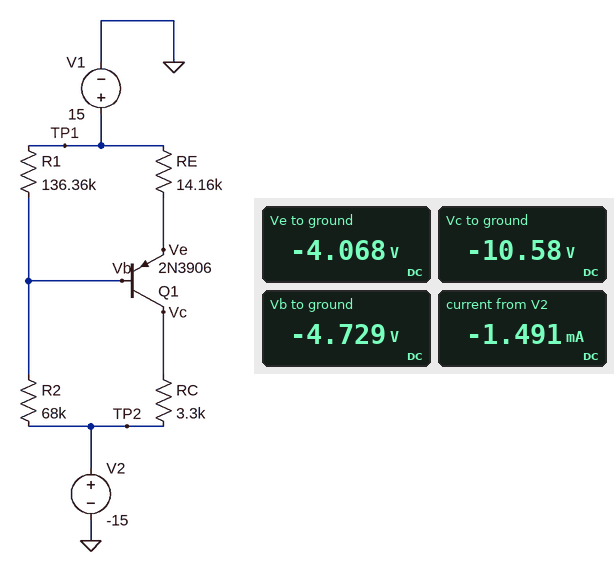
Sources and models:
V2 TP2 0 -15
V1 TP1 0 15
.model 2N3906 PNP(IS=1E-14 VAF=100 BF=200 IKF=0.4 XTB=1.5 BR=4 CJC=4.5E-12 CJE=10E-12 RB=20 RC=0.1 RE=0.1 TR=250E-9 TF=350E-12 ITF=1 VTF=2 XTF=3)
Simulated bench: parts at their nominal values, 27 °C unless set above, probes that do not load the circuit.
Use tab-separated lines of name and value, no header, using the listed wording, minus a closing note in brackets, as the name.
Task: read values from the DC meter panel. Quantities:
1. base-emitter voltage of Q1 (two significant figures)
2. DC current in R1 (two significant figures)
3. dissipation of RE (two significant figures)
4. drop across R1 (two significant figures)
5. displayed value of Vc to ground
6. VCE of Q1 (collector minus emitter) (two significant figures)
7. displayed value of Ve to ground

base-emitter voltage of Q1	-660 mV
DC current in R1	140 µA
dissipation of RE	26 mW
drop across R1	20 V
displayed value of Vc to ground	-10.58 V
VCE of Q1 (collector minus emitter)	-6.5 V
displayed value of Ve to ground	-4.068 V
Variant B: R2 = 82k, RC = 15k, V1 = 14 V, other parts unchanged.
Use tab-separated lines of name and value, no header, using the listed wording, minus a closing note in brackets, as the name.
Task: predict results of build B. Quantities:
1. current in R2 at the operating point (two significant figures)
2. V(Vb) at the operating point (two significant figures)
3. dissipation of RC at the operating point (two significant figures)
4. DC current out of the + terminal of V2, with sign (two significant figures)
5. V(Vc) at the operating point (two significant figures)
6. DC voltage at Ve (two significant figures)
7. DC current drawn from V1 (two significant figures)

current in R2 at the operating point	170 µA
V(Vb) at the operating point	-1.1 V
dissipation of RC at the operating point	14 mW
DC current out of the + terminal of V2, with sign	-1.1 mA
V(Vc) at the operating point	-530 mV
DC voltage at Ve	-480 mV
DC current drawn from V1	1.1 mA
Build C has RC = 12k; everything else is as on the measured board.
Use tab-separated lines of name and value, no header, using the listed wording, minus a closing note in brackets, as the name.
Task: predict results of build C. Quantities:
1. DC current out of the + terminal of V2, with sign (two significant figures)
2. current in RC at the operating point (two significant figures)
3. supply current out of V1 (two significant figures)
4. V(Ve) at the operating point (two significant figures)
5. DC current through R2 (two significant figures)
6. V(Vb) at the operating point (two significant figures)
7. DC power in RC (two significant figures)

DC current out of the + terminal of V2, with sign	-1.3 mA
current in RC at the operating point	1.1 mA
supply current out of V1	1.3 mA
V(Ve) at the operating point	-1.6 V
DC current through R2	190 µA
V(Vb) at the operating point	-2.3 V
DC power in RC	15 mW
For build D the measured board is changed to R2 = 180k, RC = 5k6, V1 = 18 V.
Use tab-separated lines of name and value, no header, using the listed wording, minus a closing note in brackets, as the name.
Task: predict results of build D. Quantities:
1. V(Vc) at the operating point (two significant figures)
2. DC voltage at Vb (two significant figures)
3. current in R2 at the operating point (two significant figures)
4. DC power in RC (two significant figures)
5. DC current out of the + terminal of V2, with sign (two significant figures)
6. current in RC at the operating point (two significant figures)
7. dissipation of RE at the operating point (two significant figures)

V(Vc) at the operating point	-9.8 V
DC voltage at Vb	4.1 V
current in R2 at the operating point	110 µA
DC power in RC	4.9 mW
DC current out of the + terminal of V2, with sign	-1.0 mA
current in RC at the operating point	930 µA
dissipation of RE at the operating point	12 mW
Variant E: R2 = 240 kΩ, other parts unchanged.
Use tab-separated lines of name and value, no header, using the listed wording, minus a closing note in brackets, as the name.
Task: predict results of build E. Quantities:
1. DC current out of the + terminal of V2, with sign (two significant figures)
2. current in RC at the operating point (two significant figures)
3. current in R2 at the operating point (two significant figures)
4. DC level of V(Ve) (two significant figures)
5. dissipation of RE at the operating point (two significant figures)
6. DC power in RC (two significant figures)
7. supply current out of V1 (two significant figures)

DC current out of the + terminal of V2, with sign	-780 µA
current in RC at the operating point	700 µA
current in R2 at the operating point	81 µA
DC level of V(Ve)	5.0 V
dissipation of RE at the operating point	7.0 mW
DC power in RC	1.6 mW
supply current out of V1	780 µA
